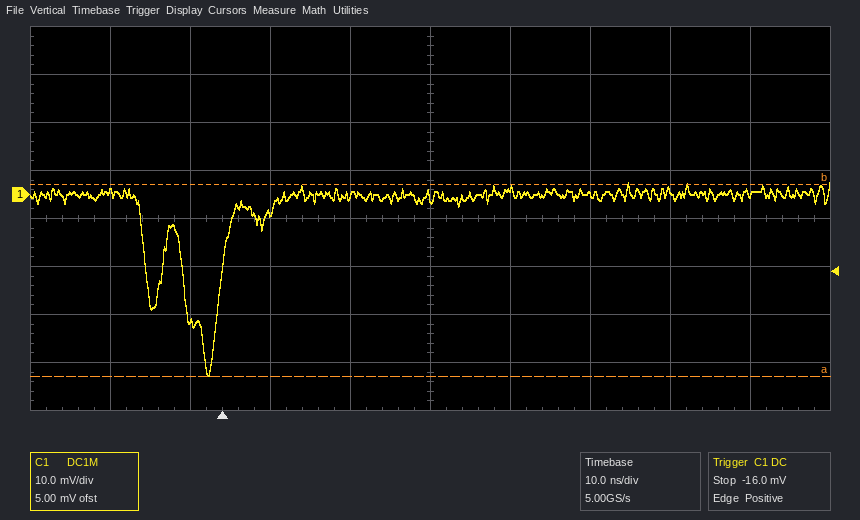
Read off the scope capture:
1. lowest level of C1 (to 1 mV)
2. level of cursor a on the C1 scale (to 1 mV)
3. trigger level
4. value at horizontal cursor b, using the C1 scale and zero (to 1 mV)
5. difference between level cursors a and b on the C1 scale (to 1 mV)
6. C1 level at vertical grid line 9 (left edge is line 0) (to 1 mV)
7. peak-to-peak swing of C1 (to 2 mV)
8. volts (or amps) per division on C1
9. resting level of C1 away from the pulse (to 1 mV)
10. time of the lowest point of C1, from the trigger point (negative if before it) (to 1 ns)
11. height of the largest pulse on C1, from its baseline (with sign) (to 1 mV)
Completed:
-38 mV
-38 mV
-16.0 mV
2 mV
40 mV
0 mV
40 mV
10 mV
0 mV
-2 ns
-38 mV
